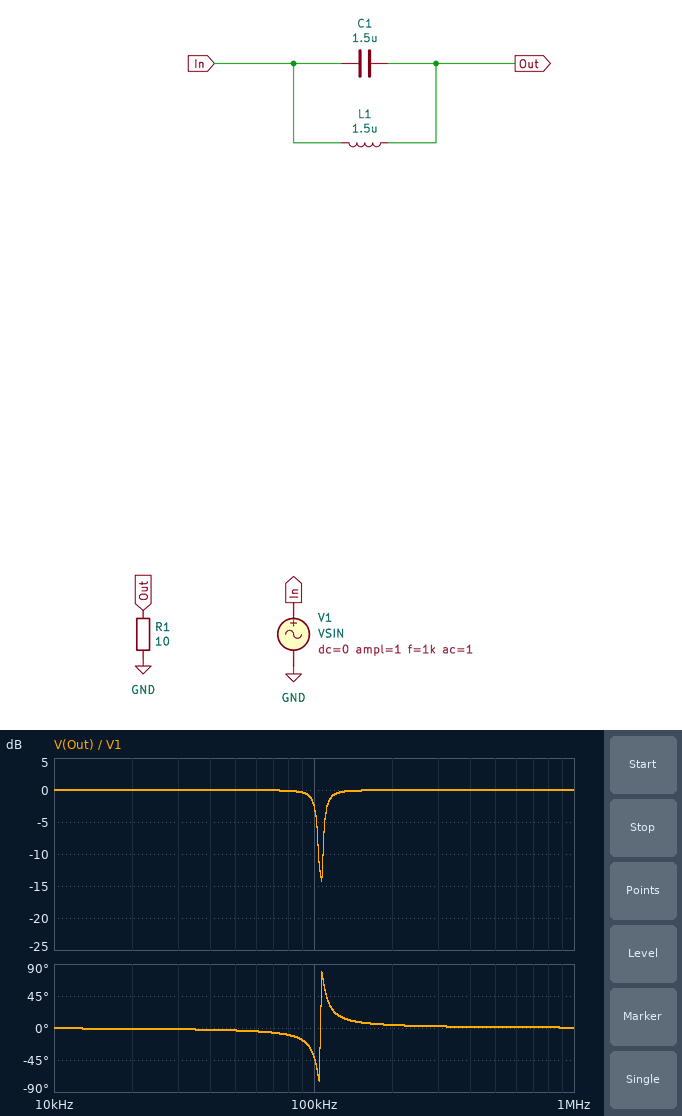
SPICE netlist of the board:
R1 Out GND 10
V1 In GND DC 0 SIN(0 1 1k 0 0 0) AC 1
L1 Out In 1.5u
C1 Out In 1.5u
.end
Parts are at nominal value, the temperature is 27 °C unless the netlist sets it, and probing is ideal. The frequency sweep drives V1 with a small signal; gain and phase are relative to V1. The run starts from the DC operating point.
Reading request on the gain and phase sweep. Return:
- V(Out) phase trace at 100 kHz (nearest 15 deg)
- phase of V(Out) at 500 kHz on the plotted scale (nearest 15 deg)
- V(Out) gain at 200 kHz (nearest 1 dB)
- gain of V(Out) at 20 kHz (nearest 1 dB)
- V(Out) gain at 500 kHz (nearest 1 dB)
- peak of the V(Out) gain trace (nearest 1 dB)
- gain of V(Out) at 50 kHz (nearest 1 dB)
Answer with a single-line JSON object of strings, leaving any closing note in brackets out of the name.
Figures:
{"V(Out) phase trace at 100 kHz": "-45 deg", "phase of V(Out) at 500 kHz on the plotted scale": "0 deg", "V(Out) gain at 200 kHz": "0 dB", "gain of V(Out) at 20 kHz": "0 dB", "V(Out) gain at 500 kHz": "0 dB", "peak of the V(Out) gain trace": "0 dB", "gain of V(Out) at 50 kHz": "0 dB"}
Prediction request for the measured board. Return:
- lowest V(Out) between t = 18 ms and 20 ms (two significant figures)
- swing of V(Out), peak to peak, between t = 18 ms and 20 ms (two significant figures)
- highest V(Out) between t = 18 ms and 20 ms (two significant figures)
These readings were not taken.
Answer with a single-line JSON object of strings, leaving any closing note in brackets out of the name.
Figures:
{"lowest V(Out) between t = 18 ms and 20 ms": "-1.0 V", "swing of V(Out), peak to peak, between t = 18 ms and 20 ms": "2.0 V", "highest V(Out) between t = 18 ms and 20 ms": "1.0 V"}
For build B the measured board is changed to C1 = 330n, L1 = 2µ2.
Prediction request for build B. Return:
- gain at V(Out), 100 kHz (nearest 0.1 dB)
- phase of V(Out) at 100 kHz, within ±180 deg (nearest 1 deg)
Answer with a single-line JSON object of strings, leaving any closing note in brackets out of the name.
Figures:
{"gain at V(Out), 100 kHz": "-0.2 dB", "phase of V(Out) at 100 kHz, within ±180 deg": "-11 deg"}
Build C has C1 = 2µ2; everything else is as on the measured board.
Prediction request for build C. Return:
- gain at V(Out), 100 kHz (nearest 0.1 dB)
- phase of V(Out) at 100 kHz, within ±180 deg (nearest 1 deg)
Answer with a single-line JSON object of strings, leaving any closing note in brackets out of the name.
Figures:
{"gain at V(Out), 100 kHz": "-0.4 dB", "phase of V(Out) at 100 kHz, within ±180 deg": "17 deg"}
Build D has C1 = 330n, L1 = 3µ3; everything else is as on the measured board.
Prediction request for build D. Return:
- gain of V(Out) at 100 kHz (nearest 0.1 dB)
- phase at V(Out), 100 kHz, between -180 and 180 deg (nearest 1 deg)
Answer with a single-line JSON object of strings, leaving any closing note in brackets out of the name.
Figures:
{"gain of V(Out) at 100 kHz": "-0.5 dB", "phase at V(Out), 100 kHz, between -180 and 180 deg": "-20 deg"}
